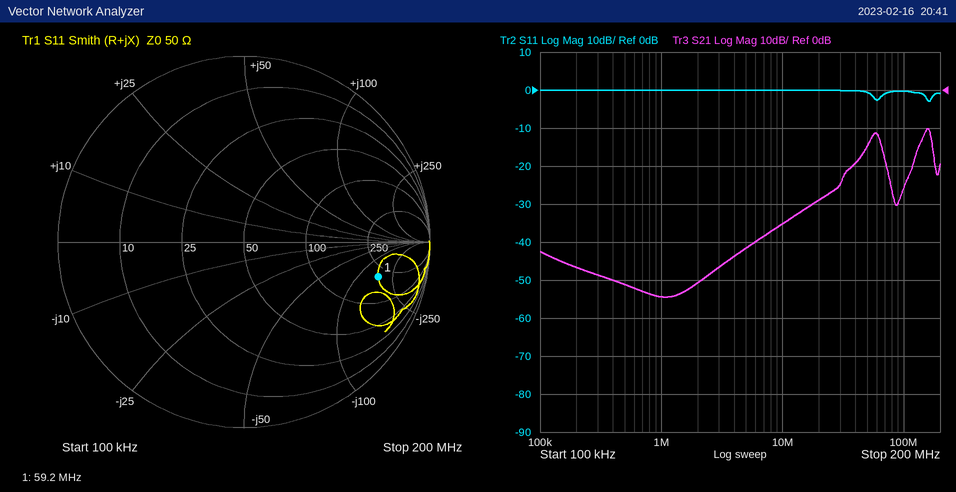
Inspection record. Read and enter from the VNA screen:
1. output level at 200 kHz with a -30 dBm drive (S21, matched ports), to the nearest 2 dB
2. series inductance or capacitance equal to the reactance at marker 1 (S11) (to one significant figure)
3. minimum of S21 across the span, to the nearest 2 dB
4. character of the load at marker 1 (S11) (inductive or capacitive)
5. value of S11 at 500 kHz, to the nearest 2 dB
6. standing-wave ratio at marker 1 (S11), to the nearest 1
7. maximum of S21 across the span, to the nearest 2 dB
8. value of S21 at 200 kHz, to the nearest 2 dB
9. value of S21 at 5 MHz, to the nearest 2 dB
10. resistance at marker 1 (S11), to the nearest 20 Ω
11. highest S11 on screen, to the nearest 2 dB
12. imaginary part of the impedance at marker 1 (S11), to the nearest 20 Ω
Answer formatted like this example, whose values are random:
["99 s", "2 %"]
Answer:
["-76 dBm", "20 pF", "-54 dB", "capacitive", "0 dB", "7", "-10 dB", "-46 dB", "-42 dB", "200 Ω", "0 dB", "-160 Ω"]
